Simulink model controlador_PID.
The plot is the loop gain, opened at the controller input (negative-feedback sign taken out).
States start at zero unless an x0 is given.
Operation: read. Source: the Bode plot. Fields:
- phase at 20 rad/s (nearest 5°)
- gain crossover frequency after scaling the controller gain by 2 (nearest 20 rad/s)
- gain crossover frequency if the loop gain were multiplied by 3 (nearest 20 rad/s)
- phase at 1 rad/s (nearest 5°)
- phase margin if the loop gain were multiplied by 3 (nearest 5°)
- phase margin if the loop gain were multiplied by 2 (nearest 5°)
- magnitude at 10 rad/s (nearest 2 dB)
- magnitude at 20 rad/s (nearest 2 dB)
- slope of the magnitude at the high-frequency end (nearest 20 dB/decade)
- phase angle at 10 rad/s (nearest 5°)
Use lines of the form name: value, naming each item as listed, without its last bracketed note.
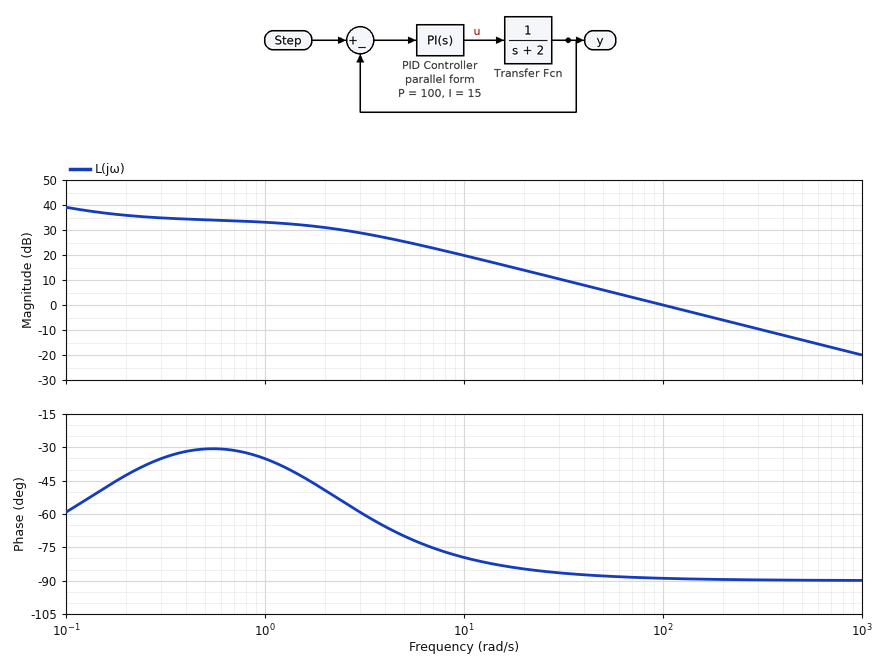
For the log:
phase at 20 rad/s: -85°
gain crossover frequency after scaling the controller gain by 2: 200 rad/s
gain crossover frequency if the loop gain were multiplied by 3: 300 rad/s
phase at 1 rad/s: -35°
phase margin if the loop gain were multiplied by 3: 90°
phase margin if the loop gain were multiplied by 2: 90°
magnitude at 10 rad/s: 20 dB
magnitude at 20 rad/s: 14 dB
slope of the magnitude at the high-frequency end: -20 dB/decade
phase angle at 10 rad/s: -80°
